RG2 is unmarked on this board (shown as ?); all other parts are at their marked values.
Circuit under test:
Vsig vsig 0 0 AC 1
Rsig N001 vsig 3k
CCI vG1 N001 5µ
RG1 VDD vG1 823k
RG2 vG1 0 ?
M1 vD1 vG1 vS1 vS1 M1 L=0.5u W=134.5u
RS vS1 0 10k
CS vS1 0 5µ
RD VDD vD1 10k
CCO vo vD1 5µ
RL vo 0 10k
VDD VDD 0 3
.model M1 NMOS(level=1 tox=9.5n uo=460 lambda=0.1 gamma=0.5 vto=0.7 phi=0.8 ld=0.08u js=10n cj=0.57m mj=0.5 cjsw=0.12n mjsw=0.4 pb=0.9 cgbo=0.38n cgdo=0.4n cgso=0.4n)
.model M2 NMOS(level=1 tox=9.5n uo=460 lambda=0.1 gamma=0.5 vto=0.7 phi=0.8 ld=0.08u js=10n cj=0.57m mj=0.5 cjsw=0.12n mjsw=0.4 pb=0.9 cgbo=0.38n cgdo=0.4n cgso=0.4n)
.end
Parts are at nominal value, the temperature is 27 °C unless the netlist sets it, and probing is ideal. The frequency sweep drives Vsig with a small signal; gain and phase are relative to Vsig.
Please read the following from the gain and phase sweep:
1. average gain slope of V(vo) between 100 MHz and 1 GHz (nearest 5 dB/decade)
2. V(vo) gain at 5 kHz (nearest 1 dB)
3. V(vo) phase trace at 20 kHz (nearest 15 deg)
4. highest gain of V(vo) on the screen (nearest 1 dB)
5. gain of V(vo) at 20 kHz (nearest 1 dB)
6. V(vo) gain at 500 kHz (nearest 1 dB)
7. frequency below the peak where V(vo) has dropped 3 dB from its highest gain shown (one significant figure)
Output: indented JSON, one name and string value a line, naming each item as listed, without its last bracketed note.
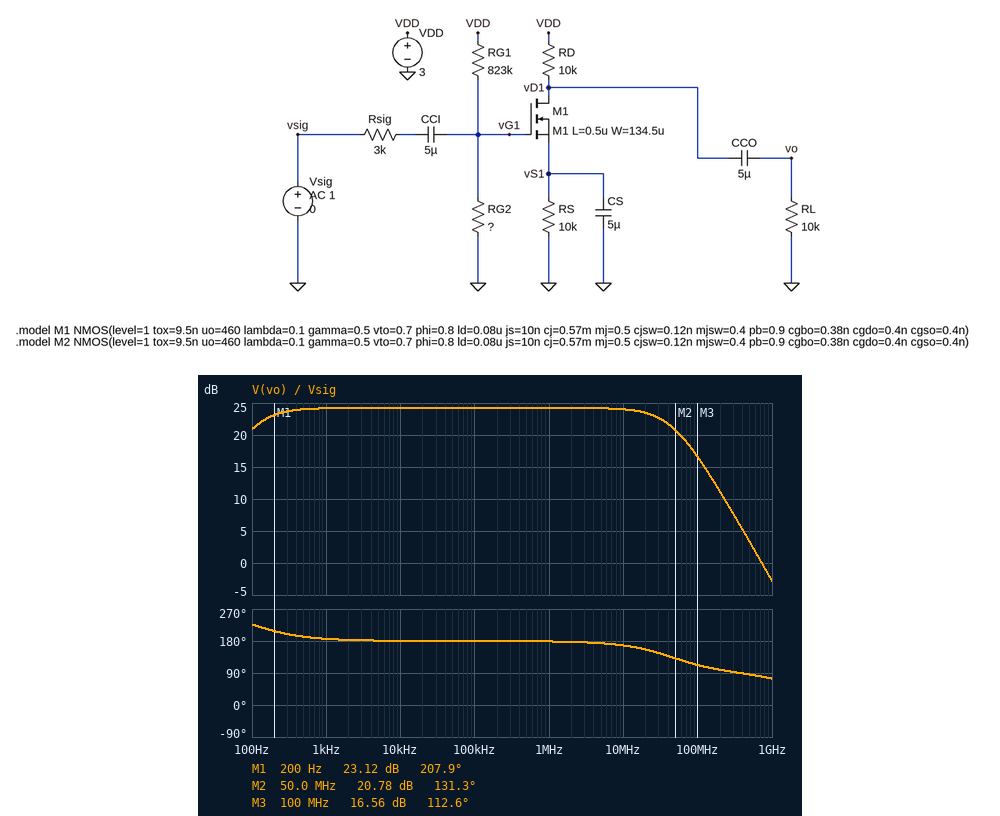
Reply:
{
  "average gain slope of V(vo) between 100 MHz and 1 GHz": "-20 dB/decade",
  "V(vo) gain at 5 kHz": "24 dB",
  "V(vo) phase trace at 20 kHz": "180 deg",
  "highest gain of V(vo) on the screen": "24 dB",
  "gain of V(vo) at 20 kHz": "24 dB",
  "V(vo) gain at 500 kHz": "24 dB",
  "frequency below the peak where V(vo) has dropped 3 dB from its highest gain shown": "100 Hz"
}
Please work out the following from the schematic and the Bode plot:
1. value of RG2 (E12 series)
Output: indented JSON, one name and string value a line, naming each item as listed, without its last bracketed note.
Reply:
{
  "value of RG2": "820 kΩ"
}
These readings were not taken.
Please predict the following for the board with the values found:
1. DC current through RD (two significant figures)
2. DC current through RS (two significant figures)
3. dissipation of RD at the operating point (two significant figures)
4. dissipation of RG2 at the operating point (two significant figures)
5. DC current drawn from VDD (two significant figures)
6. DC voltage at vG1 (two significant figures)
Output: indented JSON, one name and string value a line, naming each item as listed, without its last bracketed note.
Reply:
{
  "DC current through RD": "75 µA",
  "DC current through RS": "75 µA",
  "dissipation of RD at the operating point": "57 µW",
  "dissipation of RG2 at the operating point": "2.7 µW",
  "DC current drawn from VDD": "77 µA",
  "DC voltage at vG1": "1.5 V"
}
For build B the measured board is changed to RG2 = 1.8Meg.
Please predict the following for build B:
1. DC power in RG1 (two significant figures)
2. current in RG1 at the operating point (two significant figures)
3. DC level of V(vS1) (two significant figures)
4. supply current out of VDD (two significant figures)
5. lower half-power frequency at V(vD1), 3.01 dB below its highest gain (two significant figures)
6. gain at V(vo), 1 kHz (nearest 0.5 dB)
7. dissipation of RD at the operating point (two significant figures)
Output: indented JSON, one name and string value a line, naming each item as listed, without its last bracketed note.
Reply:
{
  "DC power in RG1": "1.1 µW",
  "current in RG1 at the operating point": "1.1 µA",
  "DC level of V(vS1)": "1.3 V",
  "supply current out of VDD": "130 µA",
  "lower half-power frequency at V(vD1), 3.01 dB below its highest gain": "130 Hz",
  "gain at V(vo), 1 kHz": "26.0 dB",
  "dissipation of RD at the operating point": "170 µW"
}
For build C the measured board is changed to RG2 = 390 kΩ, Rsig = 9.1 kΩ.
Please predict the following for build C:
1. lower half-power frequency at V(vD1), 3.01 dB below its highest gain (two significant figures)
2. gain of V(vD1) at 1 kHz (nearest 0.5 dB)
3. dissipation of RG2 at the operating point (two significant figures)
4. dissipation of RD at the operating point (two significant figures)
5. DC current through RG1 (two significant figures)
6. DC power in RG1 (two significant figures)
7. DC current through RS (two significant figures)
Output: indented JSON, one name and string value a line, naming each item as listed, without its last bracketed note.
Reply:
{
  "lower half-power frequency at V(vD1), 3.01 dB below its highest gain": "66 Hz",
  "gain of V(vD1) at 1 kHz": "19.5 dB",
  "dissipation of RG2 at the operating point": "2.4 µW",
  "dissipation of RD at the operating point": "5.8 µW",
  "DC current through RG1": "2.5 µA",
  "DC power in RG1": "5.0 µW",
  "DC current through RS": "24 µA"
}
